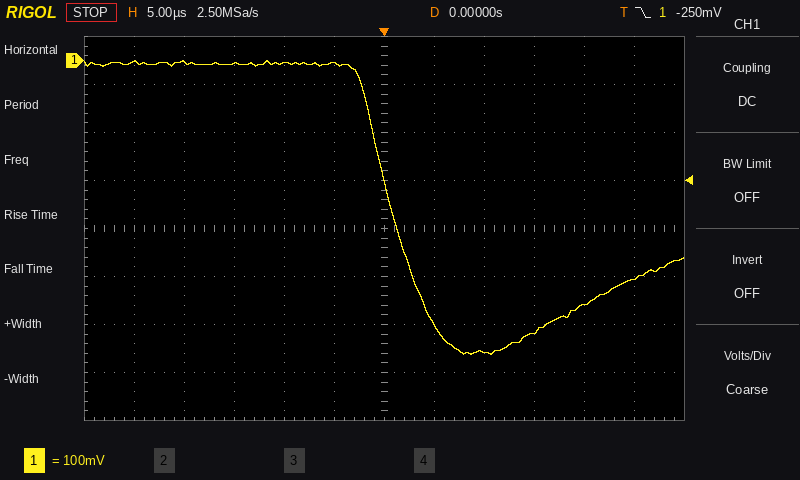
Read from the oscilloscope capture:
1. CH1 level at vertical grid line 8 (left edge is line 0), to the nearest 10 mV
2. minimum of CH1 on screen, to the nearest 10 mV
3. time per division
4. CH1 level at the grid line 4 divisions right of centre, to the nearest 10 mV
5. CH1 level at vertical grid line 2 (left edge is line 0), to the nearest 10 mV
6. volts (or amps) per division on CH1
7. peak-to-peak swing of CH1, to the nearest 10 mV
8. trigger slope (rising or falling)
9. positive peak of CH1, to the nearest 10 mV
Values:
-610 mV
-610 mV
5 µs
-510 mV
0 mV
100 mV
610 mV
falling
0 mV
